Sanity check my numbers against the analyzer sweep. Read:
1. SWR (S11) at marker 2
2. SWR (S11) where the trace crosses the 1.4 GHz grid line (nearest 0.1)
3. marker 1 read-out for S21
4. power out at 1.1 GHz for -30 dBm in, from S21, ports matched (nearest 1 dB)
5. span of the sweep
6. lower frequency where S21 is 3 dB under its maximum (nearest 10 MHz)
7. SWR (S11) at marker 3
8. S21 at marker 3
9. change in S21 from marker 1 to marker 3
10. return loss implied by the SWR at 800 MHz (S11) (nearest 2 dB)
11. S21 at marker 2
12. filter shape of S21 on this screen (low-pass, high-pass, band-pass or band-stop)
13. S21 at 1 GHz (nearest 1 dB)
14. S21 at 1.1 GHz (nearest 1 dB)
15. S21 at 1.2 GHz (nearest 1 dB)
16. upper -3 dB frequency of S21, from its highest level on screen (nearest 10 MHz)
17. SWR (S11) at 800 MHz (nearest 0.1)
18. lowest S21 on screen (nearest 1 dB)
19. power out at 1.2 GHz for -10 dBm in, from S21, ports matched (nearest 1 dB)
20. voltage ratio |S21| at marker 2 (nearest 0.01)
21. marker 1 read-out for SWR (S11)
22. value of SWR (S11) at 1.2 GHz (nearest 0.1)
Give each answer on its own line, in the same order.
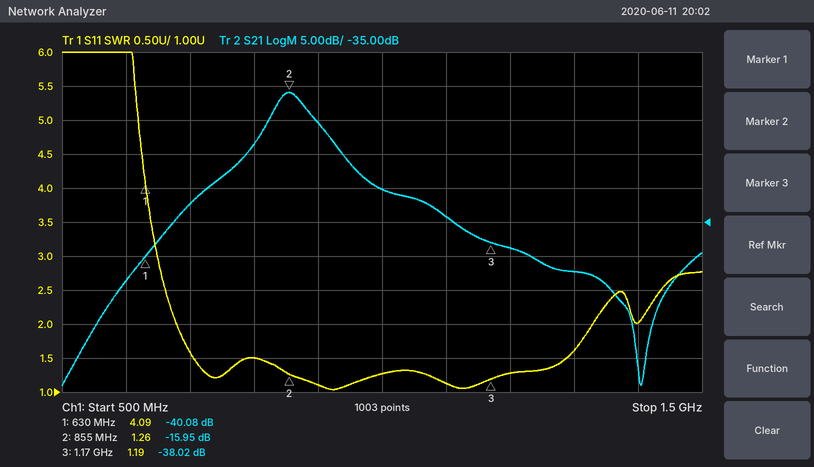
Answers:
1.26
2.0
-40.08 dB
-64 dBm
1 GHz
830 MHz
1.19
-38.02 dB
2.06 dB
14 dB
-15.95 dB
band-pass
-30 dB
-34 dB
-39 dB
890 MHz
1.5
-59 dB
-49 dBm
0.16
4.09
1.3
